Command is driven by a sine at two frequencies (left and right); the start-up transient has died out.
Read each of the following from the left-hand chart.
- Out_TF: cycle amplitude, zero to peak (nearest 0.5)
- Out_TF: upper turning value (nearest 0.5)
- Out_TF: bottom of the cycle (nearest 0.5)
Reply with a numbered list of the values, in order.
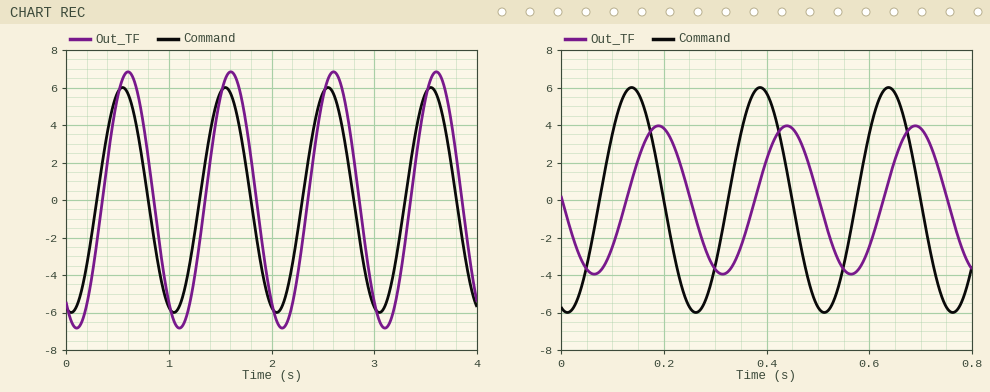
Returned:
1. 7.0
2. 7.0
3. -7.0
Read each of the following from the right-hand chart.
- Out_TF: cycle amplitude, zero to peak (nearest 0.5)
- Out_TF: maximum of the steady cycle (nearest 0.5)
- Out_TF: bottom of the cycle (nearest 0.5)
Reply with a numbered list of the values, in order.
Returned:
1. 4.0
2. 4.0
3. -4.0
